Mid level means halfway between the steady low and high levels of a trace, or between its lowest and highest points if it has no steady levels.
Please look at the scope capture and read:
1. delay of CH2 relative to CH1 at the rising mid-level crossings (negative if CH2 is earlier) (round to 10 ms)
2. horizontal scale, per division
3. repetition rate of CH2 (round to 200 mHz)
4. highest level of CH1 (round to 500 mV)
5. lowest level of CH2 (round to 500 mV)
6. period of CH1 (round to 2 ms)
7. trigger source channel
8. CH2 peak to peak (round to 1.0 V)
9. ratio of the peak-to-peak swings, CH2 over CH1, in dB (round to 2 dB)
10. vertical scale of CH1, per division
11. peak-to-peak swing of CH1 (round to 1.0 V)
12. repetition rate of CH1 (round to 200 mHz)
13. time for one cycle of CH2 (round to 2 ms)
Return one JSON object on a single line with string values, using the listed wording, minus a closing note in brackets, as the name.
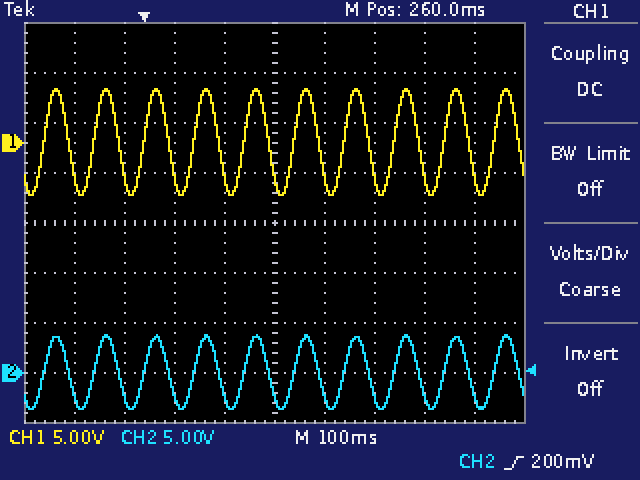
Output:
{"delay of CH2 relative to CH1 at the rising mid-level crossings (negative if CH2 is earlier)": "0 ms", "horizontal scale, per division": "100 ms", "repetition rate of CH2": "10.0 Hz", "highest level of CH1": "5.5 V", "lowest level of CH2": "-3.5 V", "period of CH1": "100 ms", "trigger source channel": "CH2", "CH2 peak to peak": "7.0 V", "ratio of the peak-to-peak swings, CH2 over CH1, in dB": "-4 dB", "vertical scale of CH1, per division": "5 V", "peak-to-peak swing of CH1": "11.0 V", "repetition rate of CH1": "10.0 Hz", "time for one cycle of CH2": "100 ms"}
